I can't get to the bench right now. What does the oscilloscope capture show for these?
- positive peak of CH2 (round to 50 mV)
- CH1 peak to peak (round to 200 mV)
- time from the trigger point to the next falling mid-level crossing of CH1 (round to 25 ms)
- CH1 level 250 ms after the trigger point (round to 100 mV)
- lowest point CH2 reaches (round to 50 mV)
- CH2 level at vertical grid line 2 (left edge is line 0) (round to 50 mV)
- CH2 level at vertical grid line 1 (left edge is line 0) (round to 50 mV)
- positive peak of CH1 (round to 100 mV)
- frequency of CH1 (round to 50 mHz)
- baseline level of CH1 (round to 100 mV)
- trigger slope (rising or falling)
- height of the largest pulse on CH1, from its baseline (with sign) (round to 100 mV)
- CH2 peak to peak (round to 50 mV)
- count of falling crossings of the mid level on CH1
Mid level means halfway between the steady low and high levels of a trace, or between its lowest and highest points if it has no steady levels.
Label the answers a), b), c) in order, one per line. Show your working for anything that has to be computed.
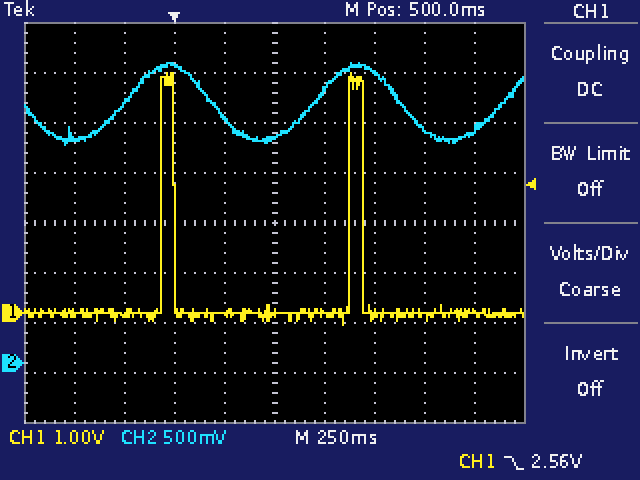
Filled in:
a) 3.00 V
b) 5.0 V
c) 950 ms
d) 0.0 V
e) 2.20 V
f) 2.60 V
g) 2.25 V
h) 4.8 V
i) 1.05 Hz
j) 0.0 V
k) falling
l) 4.8 V − (0.0 V) = +4.8 V
m) 3.00 V − (2.20 V) = 800 mV
n) 2
